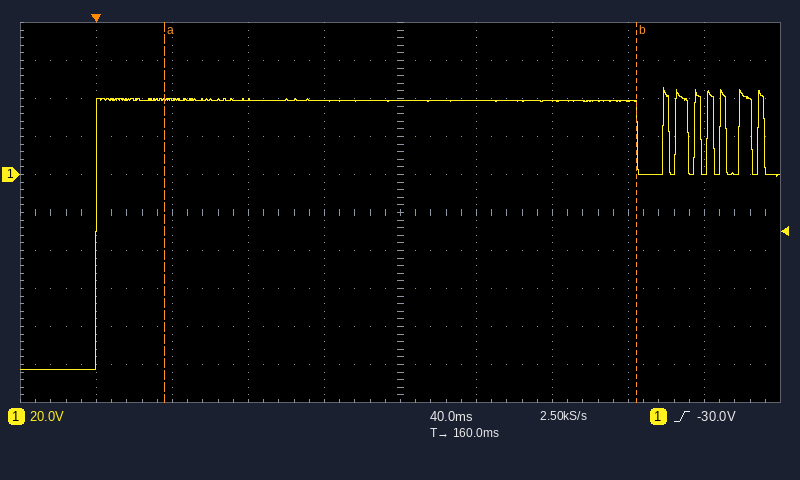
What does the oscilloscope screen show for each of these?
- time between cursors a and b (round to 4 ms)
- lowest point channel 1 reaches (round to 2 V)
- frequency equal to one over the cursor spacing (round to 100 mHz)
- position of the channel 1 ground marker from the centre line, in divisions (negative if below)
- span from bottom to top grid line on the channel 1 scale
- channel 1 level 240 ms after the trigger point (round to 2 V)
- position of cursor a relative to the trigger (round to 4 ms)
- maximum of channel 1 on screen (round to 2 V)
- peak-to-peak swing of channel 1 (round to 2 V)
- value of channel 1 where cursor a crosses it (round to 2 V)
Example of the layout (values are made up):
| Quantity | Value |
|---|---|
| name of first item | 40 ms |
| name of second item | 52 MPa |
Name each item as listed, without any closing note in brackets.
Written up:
| Quantity | Value |
|---|---|
| time between cursors a and b | 248 ms |
| lowest point channel 1 reaches | -102 V |
| frequency equal to one over the cursor spacing | 4.0 Hz |
| position of the channel 1 ground marker from the centre line, in divisions | +1.0 div |
| span from bottom to top grid line on the channel 1 scale | 200 V |
| channel 1 level 240 ms after the trigger point | 38 V |
| position of cursor a relative to the trigger | +36 ms |
| maximum of channel 1 on screen | 46 V |
| peak-to-peak swing of channel 1 | 148 V |
| value of channel 1 where cursor a crosses it | 40 V |
